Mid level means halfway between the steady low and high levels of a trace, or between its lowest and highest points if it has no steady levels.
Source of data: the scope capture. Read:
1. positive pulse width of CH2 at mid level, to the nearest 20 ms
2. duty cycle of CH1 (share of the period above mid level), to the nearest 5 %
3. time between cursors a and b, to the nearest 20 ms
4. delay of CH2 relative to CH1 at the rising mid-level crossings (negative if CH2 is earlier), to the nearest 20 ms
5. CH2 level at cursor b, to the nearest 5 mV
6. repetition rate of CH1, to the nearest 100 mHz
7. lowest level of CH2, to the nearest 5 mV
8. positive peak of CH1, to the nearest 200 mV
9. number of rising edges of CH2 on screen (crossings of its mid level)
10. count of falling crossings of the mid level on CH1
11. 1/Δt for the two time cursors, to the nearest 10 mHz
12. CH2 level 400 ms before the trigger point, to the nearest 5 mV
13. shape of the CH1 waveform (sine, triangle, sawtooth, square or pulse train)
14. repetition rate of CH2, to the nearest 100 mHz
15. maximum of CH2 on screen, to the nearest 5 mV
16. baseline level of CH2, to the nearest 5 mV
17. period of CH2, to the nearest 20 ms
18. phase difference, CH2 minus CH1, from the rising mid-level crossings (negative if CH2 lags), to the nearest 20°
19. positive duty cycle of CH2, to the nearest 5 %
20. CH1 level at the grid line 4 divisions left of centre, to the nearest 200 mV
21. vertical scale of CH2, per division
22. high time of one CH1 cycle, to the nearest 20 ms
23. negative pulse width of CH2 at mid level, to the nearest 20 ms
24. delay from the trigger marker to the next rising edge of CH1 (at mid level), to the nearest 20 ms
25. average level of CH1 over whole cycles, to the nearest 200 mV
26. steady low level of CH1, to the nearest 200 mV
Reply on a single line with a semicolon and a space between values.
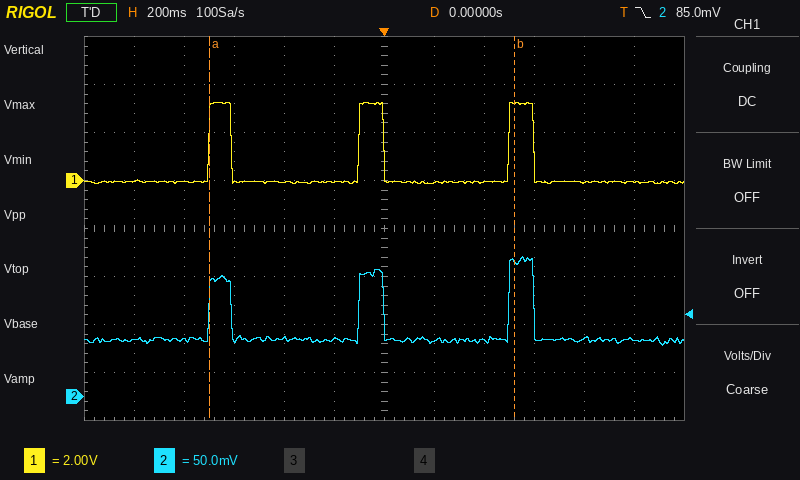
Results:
100 ms; 15 %; 1.22 s; 0 ms; 140 mV; 1.7 Hz; 55 mV; 3.2 V; 3; 3; 820 mHz; 60 mV; pulse train; 1.7 Hz; 145 mV; 60 mV; 600 ms; 0°; 15 %; 0.0 V; 50 mV; 100 ms; 500 ms; 500 ms; 400 mV; 0.0 V
